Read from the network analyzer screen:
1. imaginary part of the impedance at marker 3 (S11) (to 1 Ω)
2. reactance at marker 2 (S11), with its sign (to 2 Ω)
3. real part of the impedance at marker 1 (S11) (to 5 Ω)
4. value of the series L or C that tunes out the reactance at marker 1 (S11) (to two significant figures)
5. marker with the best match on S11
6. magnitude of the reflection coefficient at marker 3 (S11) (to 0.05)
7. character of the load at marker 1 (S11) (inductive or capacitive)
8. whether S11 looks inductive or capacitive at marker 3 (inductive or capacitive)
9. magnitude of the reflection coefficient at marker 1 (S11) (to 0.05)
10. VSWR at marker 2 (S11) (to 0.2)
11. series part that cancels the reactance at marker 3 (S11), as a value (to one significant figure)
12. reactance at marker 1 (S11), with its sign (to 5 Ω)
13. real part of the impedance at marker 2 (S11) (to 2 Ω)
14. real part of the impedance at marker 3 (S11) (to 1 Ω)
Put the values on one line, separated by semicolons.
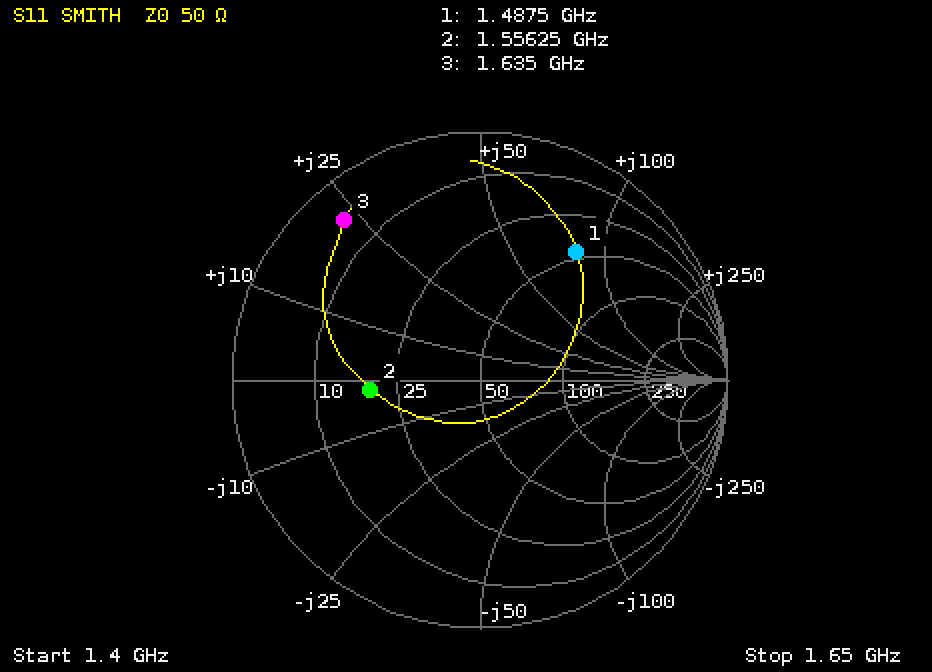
+23 Ω; -2 Ω; 45 Ω; 1.3 pF; marker 2; 0.85; inductive; inductive; 0.65; 2.6; 4 pF; +80 Ω; 20 Ω; 5 Ω
